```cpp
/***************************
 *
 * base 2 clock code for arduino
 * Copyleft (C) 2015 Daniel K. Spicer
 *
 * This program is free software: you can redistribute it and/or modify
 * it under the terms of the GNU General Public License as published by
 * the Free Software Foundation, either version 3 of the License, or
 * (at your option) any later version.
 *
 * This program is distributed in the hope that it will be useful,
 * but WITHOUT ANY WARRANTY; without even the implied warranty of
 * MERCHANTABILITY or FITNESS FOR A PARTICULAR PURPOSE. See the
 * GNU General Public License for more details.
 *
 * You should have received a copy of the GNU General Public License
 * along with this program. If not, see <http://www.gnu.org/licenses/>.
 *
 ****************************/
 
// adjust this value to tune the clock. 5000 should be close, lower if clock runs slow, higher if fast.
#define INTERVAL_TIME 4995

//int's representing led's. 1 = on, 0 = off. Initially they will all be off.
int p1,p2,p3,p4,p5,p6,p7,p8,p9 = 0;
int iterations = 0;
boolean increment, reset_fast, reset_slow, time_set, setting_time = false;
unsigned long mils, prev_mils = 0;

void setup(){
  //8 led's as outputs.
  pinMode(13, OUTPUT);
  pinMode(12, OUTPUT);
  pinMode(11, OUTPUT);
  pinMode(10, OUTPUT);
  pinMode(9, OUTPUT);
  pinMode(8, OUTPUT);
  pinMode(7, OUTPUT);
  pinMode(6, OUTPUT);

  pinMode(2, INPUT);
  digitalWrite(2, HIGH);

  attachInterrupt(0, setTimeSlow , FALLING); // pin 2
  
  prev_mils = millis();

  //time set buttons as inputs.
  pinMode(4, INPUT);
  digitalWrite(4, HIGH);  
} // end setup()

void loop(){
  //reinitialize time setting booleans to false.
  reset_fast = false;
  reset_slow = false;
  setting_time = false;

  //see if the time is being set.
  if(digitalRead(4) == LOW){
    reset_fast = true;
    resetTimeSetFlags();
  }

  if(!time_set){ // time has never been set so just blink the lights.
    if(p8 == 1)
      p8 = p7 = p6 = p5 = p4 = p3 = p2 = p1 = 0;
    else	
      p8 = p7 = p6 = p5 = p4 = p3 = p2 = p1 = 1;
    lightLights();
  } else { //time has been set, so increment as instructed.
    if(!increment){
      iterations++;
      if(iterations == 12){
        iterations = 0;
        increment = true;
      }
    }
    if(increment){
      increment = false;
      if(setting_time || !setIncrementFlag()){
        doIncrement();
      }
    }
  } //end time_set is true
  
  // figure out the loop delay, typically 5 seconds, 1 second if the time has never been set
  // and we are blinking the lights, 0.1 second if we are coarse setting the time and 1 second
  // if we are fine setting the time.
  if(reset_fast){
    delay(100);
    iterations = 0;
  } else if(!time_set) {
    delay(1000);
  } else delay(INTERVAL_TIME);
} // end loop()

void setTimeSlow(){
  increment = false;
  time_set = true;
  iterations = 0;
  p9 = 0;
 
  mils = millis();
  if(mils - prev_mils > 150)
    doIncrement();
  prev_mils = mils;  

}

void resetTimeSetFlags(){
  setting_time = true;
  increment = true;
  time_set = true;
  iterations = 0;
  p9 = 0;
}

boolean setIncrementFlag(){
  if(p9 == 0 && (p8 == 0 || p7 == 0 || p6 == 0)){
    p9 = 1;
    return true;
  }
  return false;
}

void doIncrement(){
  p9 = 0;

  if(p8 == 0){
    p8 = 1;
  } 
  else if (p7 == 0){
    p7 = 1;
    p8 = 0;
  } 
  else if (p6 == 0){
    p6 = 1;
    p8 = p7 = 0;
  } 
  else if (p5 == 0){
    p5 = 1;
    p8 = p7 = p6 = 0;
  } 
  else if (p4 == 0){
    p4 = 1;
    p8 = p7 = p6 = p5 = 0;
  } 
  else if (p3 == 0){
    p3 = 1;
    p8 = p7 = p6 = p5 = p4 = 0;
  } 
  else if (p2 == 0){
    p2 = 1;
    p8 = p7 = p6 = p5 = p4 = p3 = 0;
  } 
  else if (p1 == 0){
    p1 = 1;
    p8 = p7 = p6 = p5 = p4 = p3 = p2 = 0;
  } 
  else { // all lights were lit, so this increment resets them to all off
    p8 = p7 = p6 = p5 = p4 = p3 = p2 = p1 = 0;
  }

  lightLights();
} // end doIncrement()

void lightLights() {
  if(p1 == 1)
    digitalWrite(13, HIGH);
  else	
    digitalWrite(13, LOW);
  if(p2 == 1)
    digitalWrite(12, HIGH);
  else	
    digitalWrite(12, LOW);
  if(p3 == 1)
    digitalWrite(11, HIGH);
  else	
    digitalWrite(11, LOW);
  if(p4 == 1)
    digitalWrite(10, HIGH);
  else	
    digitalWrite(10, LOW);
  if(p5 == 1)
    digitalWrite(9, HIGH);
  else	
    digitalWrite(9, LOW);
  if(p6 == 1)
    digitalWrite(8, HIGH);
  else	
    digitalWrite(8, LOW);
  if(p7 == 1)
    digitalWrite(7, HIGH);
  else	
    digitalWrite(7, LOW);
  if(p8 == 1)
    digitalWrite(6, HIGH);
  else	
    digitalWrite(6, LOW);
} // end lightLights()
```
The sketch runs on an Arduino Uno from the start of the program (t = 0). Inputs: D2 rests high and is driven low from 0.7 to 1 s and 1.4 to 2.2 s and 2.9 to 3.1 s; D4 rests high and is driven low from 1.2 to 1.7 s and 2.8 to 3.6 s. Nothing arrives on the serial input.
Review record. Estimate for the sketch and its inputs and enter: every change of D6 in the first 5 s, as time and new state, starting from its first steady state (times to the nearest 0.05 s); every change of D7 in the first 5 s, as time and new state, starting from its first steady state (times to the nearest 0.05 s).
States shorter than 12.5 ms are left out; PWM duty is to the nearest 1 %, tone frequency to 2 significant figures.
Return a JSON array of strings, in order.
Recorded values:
["0 s high; 0.7 s low; 1.4 s high; 2.9 s low", "0 s high; 0.7 s low; 2.9 s high"]
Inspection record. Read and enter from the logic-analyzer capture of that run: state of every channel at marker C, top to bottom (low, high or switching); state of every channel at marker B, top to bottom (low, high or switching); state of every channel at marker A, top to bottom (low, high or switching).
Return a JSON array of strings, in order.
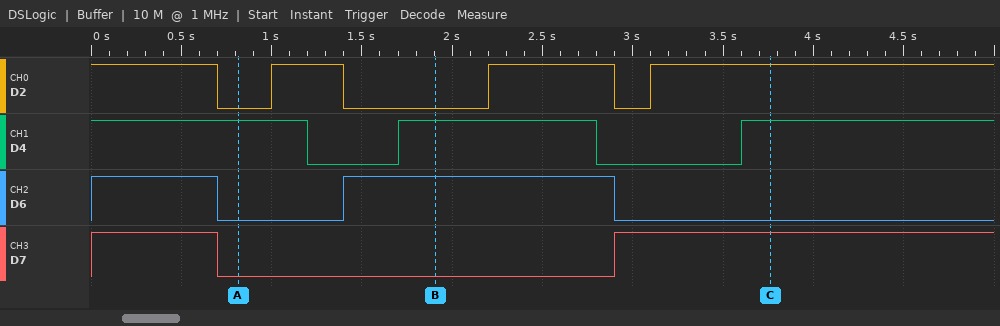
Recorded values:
["D2 high, D4 high, D6 low, D7 high", "D2 low, D4 high, D6 high, D7 low", "D2 low, D4 high, D6 low, D7 low"]
